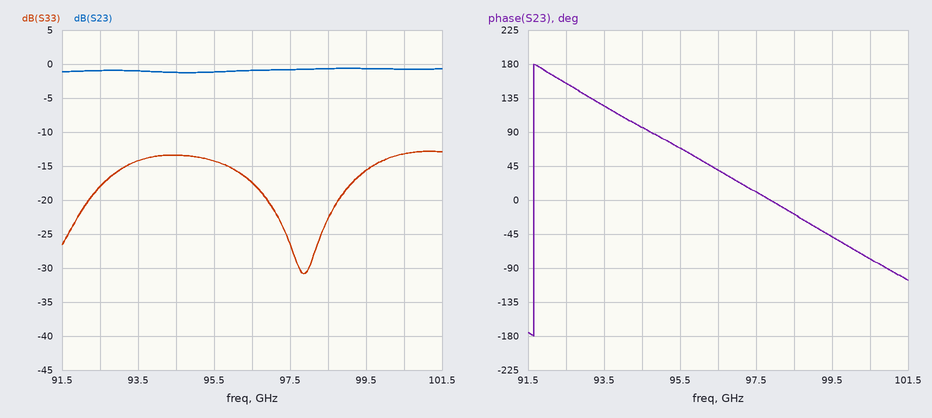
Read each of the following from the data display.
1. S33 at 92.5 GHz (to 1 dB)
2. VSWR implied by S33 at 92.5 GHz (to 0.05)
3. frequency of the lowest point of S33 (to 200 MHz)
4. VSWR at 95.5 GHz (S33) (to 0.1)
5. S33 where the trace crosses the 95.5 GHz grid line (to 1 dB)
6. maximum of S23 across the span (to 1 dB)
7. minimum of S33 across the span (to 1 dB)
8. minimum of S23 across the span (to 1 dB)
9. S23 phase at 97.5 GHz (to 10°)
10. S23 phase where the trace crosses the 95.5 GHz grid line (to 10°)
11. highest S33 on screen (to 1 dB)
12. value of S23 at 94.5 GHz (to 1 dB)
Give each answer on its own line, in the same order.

-18 dB
1.30
97.8 GHz
1.5
-14 dB
-1 dB
-31 dB
-1 dB
10°
70°
-13 dB
-1 dB
